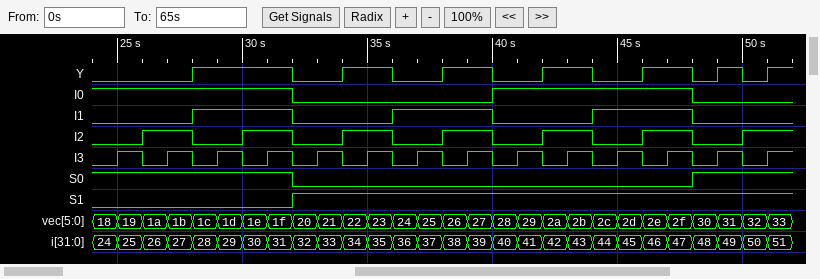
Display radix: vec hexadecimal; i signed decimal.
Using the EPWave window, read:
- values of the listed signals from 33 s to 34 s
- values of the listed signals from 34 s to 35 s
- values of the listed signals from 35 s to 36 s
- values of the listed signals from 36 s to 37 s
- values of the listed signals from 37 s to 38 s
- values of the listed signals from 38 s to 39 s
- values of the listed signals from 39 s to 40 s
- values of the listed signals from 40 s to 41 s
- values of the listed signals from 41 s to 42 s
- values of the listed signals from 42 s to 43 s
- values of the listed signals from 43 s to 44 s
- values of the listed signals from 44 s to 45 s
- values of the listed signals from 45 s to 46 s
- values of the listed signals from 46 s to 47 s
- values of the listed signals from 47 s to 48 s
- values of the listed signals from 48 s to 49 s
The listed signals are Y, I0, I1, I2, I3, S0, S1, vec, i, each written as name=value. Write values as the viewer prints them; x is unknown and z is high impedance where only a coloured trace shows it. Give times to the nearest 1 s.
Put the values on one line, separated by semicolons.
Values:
Y=0, I0=0, I1=0, I2=0, I3=1, S0=0, S1=1, vec=21, i=33; Y=1, I0=0, I1=0, I2=1, I3=0, S0=0, S1=1, vec=22, i=34; Y=1, I0=0, I1=0, I2=1, I3=1, S0=0, S1=1, vec=23, i=35; Y=0, I0=0, I1=1, I2=0, I3=0, S0=0, S1=1, vec=24, i=36; Y=0, I0=0, I1=1, I2=0, I3=1, S0=0, S1=1, vec=25, i=37; Y=1, I0=0, I1=1, I2=1, I3=0, S0=0, S1=1, vec=26, i=38; Y=1, I0=0, I1=1, I2=1, I3=1, S0=0, S1=1, vec=27, i=39; Y=0, I0=1, I1=0, I2=0, I3=0, S0=0, S1=1, vec=28, i=40; Y=0, I0=1, I1=0, I2=0, I3=1, S0=0, S1=1, vec=29, i=41; Y=1, I0=1, I1=0, I2=1, I3=0, S0=0, S1=1, vec=2a, i=42; Y=1, I0=1, I1=0, I2=1, I3=1, S0=0, S1=1, vec=2b, i=43; Y=0, I0=1, I1=1, I2=0, I3=0, S0=0, S1=1, vec=2c, i=44; Y=0, I0=1, I1=1, I2=0, I3=1, S0=0, S1=1, vec=2d, i=45; Y=1, I0=1, I1=1, I2=1, I3=0, S0=0, S1=1, vec=2e, i=46; Y=1, I0=1, I1=1, I2=1, I3=1, S0=0, S1=1, vec=2f, i=47; Y=0, I0=0, I1=0, I2=0, I3=0, S0=1, S1=1, vec=30, i=48
